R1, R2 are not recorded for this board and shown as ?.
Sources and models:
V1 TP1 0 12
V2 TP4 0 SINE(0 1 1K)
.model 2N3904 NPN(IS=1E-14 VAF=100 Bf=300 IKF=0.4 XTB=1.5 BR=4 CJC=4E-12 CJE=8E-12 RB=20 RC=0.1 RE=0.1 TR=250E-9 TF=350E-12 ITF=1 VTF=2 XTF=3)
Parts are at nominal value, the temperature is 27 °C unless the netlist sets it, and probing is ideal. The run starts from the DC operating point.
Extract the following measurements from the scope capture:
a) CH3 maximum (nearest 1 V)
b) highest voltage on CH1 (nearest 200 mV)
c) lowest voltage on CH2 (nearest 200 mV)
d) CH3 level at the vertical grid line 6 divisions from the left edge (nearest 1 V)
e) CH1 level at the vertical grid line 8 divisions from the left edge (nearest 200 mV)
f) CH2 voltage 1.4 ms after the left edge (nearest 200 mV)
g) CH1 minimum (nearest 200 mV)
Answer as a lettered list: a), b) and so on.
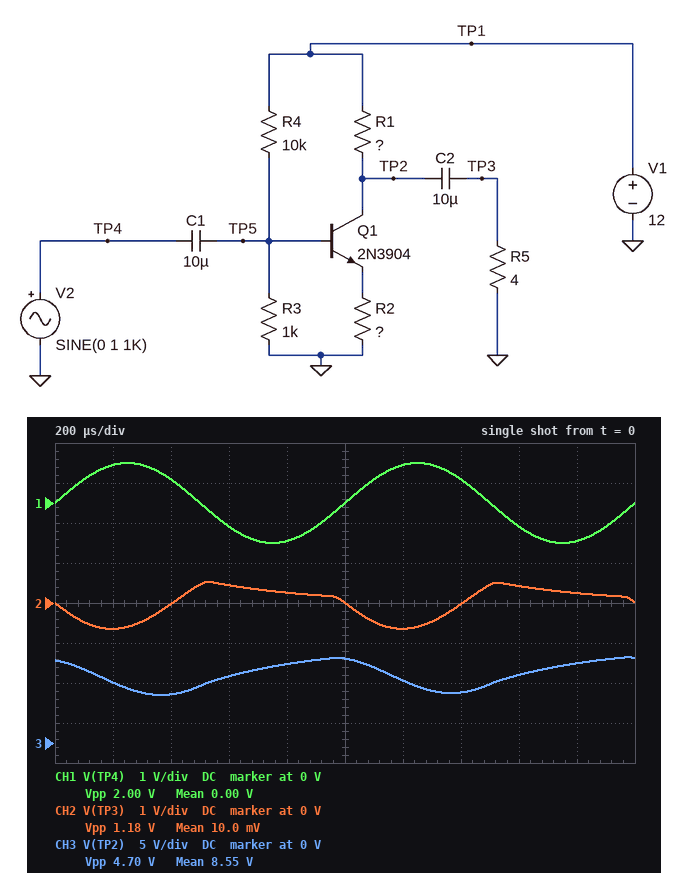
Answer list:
a) 11 V
b) 1.0 V
c) -600 mV
d) 8 V
e) -600 mV
f) 0 V
g) -1.0 V
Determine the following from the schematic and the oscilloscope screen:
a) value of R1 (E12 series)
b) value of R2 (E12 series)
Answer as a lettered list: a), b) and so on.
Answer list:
a) 33 Ω
b) 3.3 Ω
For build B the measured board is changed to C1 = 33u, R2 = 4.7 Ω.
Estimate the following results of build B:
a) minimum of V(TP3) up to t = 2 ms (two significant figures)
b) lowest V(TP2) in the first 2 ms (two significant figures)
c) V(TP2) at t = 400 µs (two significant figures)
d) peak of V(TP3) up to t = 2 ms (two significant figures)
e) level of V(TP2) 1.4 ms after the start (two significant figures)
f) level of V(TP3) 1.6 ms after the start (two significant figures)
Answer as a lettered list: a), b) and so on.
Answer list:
a) -490 mV
b) 7.3 V
c) 7.4 V
d) 410 mV
e) 7.5 V
f) 350 mV
